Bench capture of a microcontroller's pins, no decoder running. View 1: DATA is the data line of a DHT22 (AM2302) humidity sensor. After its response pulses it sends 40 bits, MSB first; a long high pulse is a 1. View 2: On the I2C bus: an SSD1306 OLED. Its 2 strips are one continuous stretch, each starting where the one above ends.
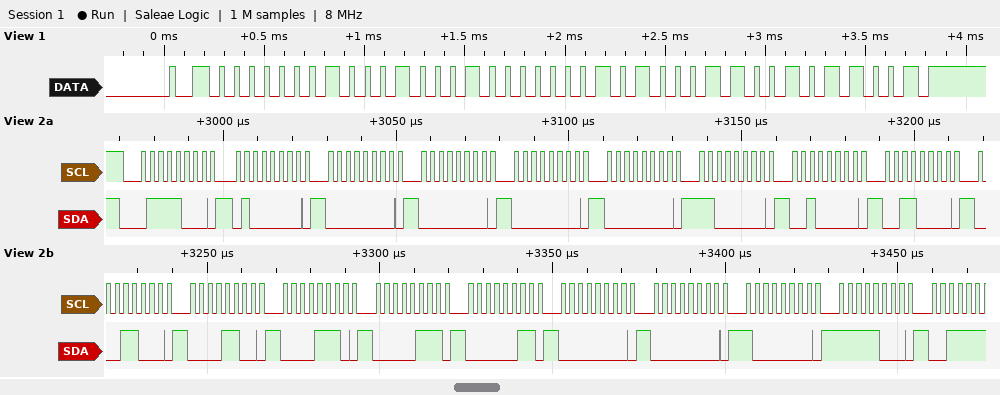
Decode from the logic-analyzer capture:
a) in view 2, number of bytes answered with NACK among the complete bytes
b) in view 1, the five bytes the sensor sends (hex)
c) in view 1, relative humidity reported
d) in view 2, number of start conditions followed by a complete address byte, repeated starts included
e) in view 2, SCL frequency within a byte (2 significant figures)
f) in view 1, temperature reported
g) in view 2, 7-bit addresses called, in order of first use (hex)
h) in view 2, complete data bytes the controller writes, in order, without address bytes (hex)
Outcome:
0
01 11 01 46 59
27.3 %
1
400 kHz
32.6 °C
0x3C
40 00 00 00 00 C0 20 30 18 0C 0E 07 03 00 00 80 F8
